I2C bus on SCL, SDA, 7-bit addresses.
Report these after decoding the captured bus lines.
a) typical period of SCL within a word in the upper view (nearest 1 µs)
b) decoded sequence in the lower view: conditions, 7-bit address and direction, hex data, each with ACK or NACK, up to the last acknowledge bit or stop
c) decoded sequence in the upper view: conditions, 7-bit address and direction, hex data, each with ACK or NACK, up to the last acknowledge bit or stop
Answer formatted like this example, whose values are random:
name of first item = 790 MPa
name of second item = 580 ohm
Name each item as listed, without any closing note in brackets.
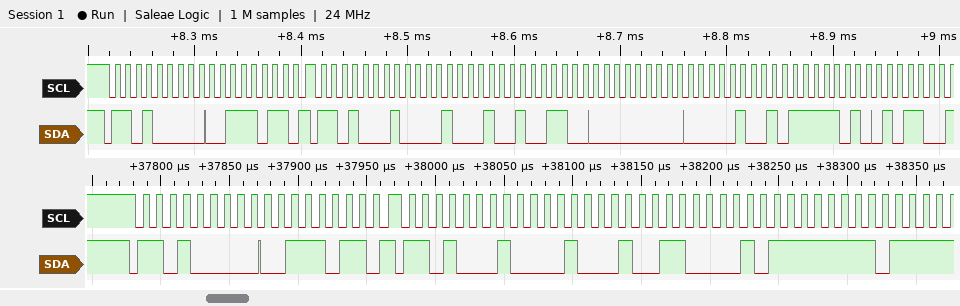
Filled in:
typical period of SCL within a word in the upper view = 10 µs
decoded sequence in the lower view: conditions, 7-bit address and direction, hex data, each with ACK or NACK, up to the last acknowledge bit or stop = start, address 68 write ACK, 3B ACK, repeated start, address 68 read ACK, 11 ACK, 61 ACK, FF ACK
decoded sequence in the upper view: conditions, 7-bit address and direction, hex data, each with ACK or NACK, up to the last acknowledge bit or stop = start, address 68 write ACK, 3B ACK, repeated start, address 68 read ACK, 11 ACK, 4C ACK, 00 ACK, 09 ACK, FA ACK
